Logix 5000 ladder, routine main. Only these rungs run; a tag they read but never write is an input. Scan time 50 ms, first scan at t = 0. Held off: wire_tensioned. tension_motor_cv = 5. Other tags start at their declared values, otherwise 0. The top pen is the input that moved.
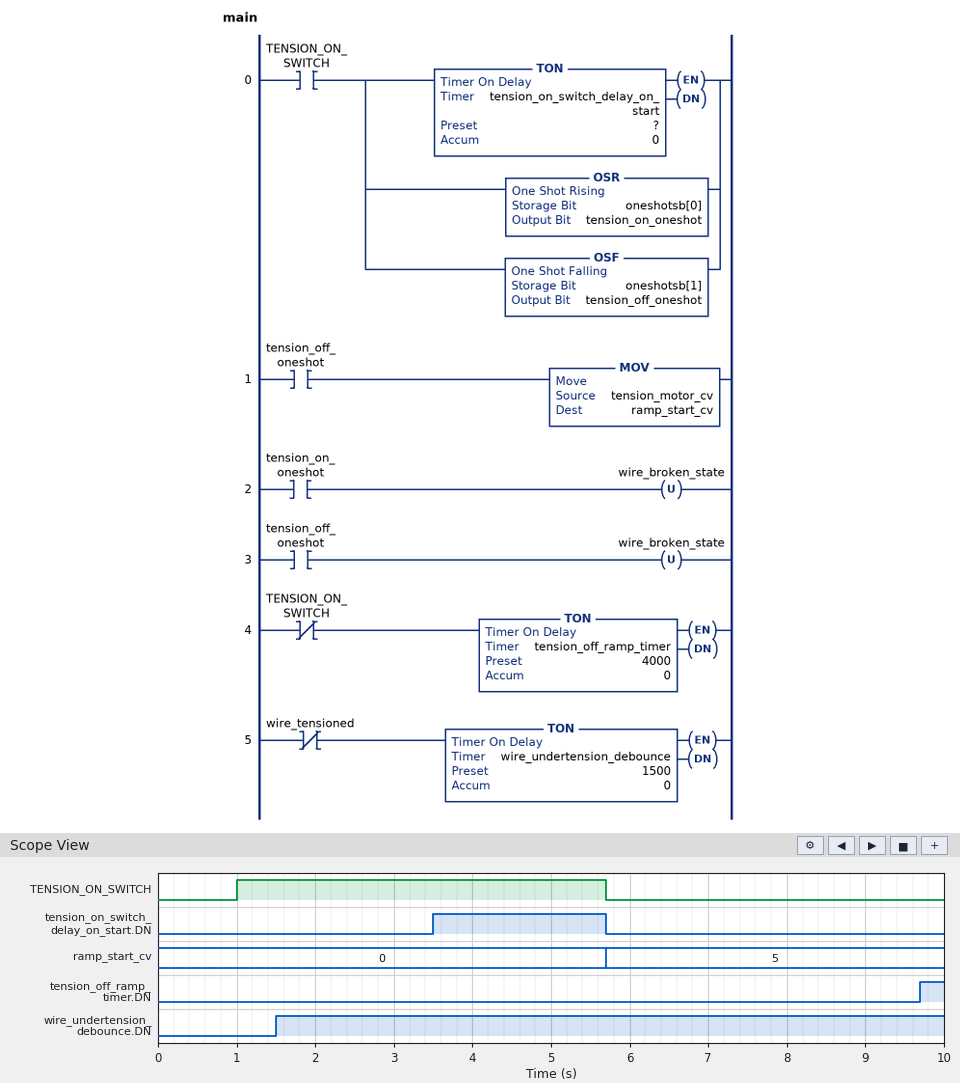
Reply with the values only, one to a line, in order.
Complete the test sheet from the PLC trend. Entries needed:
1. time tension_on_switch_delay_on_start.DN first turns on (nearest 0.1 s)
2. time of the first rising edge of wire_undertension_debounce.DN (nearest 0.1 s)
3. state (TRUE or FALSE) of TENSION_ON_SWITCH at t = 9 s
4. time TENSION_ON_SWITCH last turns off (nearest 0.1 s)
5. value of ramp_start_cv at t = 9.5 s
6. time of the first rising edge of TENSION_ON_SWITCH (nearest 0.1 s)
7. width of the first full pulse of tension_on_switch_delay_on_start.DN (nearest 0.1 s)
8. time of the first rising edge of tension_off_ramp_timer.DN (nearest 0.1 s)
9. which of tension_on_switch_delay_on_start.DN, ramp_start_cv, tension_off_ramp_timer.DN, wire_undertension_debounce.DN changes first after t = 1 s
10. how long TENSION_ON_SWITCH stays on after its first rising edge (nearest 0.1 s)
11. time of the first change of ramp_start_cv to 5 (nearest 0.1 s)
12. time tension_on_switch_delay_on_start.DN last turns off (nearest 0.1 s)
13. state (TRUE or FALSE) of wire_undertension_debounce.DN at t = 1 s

3.5 s
1.5 s
FALSE
5.7 s
5
1.0 s
2.2 s
9.7 s
wire_undertension_debounce.DN
4.7 s
5.7 s
5.7 s
FALSE
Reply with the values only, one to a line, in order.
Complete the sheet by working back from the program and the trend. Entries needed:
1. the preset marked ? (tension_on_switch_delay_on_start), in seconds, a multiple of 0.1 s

2.5 s
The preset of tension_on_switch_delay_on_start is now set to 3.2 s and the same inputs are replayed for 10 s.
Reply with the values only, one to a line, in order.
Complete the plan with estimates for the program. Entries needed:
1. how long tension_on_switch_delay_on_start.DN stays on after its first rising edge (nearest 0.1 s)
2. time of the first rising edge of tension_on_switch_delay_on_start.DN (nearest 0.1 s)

1.5 s
4.2 s
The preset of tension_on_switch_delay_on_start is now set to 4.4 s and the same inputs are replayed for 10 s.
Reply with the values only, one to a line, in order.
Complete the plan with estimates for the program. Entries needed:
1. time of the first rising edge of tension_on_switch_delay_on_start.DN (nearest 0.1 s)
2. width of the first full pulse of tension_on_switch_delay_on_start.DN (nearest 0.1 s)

5.4 s
0.3 s
